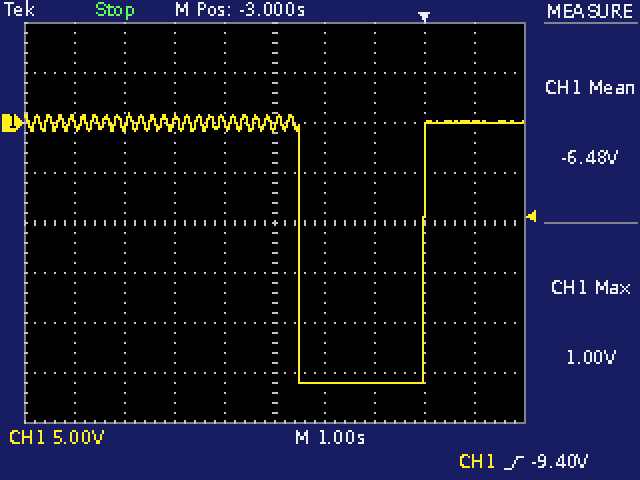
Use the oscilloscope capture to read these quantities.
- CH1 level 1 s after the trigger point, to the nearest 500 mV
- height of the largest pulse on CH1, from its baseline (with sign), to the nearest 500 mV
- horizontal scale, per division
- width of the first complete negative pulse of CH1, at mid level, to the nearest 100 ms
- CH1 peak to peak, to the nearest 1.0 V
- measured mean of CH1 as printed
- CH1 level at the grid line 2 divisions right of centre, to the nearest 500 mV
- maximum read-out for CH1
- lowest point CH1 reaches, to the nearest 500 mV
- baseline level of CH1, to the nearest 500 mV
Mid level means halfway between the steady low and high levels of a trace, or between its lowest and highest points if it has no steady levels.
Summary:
0.0 V
-26.0 V
1 s
2.5 s
27.0 V
-6.48 V
-26.0 V
1.00 V
-26.0 V
0.0 V
